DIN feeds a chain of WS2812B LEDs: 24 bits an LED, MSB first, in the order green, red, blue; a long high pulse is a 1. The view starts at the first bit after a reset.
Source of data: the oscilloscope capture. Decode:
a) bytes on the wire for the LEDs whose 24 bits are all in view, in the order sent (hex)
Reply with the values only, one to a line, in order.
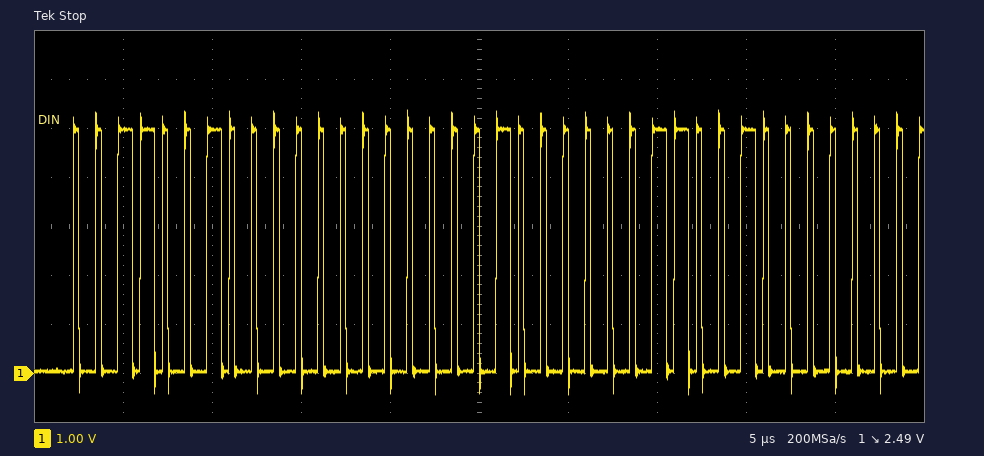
32 00 10
